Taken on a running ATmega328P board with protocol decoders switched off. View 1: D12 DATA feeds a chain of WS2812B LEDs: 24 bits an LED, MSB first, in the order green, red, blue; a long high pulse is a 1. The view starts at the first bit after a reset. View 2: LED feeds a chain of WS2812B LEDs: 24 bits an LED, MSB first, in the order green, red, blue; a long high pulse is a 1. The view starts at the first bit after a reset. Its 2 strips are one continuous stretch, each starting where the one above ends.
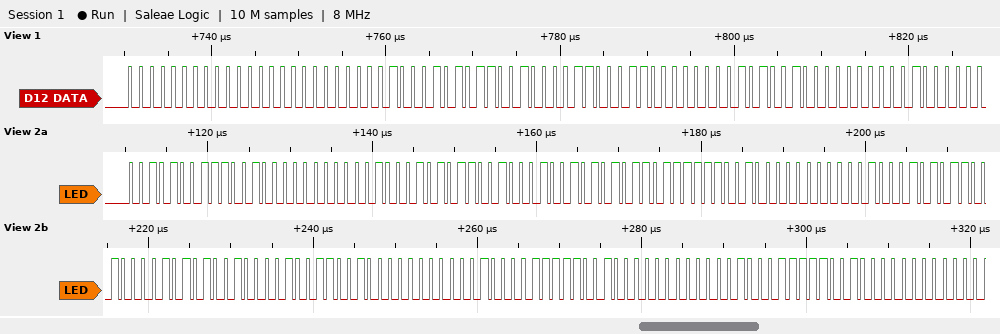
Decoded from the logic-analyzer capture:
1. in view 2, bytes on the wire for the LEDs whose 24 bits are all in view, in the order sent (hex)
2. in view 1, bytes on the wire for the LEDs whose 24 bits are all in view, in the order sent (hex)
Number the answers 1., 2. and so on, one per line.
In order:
1. 29 C8 00 8A C8 95 6F C8 00 8A C8 54 84 C8 00 87 C8 00 47 C8 00
2. 00 00 00 8A C8 63 00 A4 00
